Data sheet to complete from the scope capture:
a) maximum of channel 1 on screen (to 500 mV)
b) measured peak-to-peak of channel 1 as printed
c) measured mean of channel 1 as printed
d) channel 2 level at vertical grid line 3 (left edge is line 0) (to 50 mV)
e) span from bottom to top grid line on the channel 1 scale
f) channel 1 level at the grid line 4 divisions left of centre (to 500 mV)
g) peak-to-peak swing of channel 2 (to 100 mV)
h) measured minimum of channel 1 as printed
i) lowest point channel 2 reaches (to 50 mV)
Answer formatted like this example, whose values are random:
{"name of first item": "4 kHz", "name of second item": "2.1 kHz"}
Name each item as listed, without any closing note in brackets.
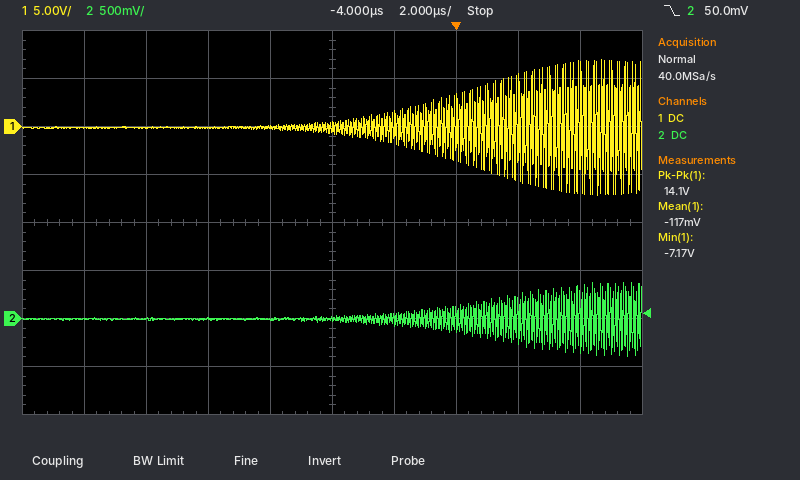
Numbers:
{"maximum of channel 1 on screen": "7.0 V", "measured peak-to-peak of channel 1 as printed": "14.1 V", "measured mean of channel 1 as printed": "-117 mV", "channel 2 level at vertical grid line 3 (left edge is line 0)": "0 mV", "span from bottom to top grid line on the channel 1 scale": "40 V", "channel 1 level at the grid line 4 divisions left of centre": "0.0 V", "peak-to-peak swing of channel 2": "800 mV", "measured minimum of channel 1 as printed": "-7.17 V", "lowest point channel 2 reaches": "-400 mV"}
